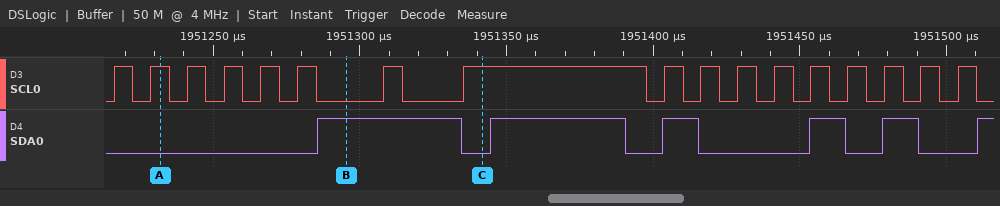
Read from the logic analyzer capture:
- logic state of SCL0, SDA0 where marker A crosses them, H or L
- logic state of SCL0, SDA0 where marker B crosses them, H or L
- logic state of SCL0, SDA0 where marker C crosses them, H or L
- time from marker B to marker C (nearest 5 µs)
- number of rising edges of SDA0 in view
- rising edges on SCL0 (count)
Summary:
SCL0=H, SDA0=L
SCL0=L, SDA0=H
SCL0=H, SDA0=L
45 µs
6
17
